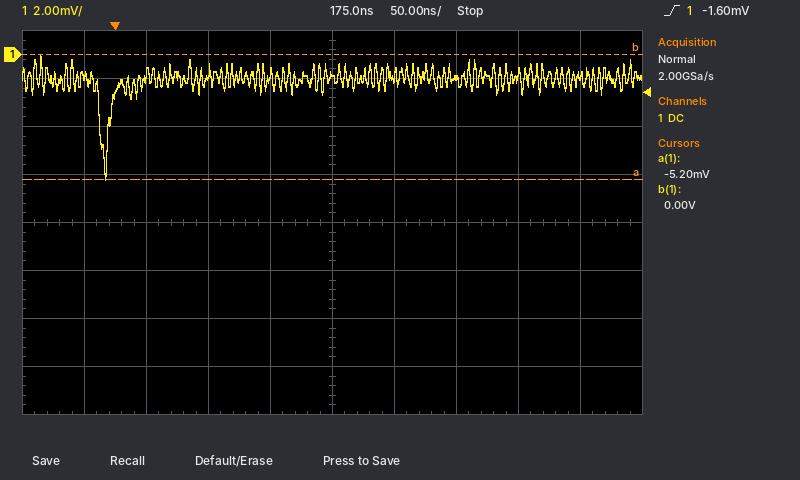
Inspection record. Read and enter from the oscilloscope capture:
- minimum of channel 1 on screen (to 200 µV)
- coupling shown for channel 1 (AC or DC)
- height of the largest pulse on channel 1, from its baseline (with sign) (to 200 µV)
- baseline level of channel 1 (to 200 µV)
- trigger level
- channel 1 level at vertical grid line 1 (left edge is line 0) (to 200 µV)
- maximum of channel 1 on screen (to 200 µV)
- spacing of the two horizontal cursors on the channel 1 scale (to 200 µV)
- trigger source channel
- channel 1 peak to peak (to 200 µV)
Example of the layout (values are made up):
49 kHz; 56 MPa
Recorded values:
-5.2 mV; DC; -4.2 mV; -1.0 mV; -1.60 mV; -800 µV; 0.0 mV; 5.2 mV; channel 1; 5.2 mV
